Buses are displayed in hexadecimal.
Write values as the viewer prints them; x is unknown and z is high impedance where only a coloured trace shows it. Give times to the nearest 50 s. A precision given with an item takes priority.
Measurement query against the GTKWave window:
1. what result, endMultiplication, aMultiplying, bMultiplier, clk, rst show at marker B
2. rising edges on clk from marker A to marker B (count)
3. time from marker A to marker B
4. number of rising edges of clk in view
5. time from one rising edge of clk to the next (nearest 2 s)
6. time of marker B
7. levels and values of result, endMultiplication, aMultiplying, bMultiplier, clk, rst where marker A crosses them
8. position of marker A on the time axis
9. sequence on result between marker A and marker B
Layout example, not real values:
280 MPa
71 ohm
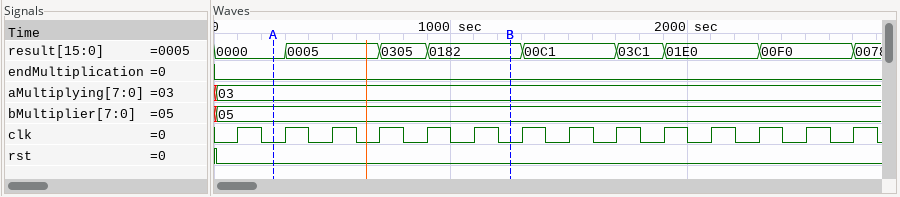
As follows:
result=0182, endMultiplication=0, aMultiplying=03, bMultiplier=05, clk=0, rst=0
5
1000 s
14
200 s
1250 s
result=0000, endMultiplication=0, aMultiplying=03, bMultiplier=05, clk=0, rst=0
250 s
0000, 0005, 0305, 0182
